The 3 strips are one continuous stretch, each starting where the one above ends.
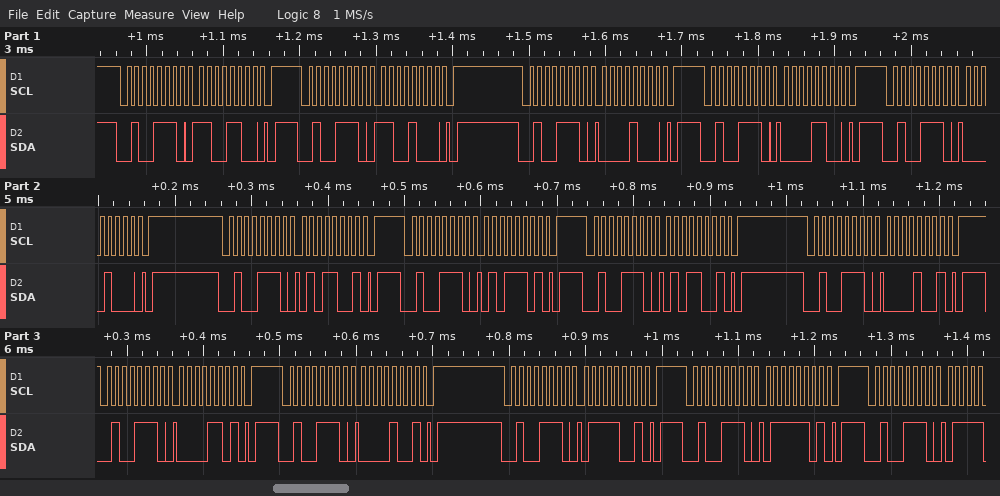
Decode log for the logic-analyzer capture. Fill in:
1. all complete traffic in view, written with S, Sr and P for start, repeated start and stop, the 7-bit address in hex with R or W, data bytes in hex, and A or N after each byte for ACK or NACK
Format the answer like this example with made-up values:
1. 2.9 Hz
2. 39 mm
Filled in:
1. S 27W A CC A P S 27W A C8 A P S 27W A 08 A P S 27W A 0C A P S 27W A 08 A P S 27W A 59 A P S 27W A 5D A P S 27W A 59 A P S 27W A 09 A P S 27W A 0D A P S 27W A 09 A P S 27W A 79 A P S 27W A 7D A P S 27W A
